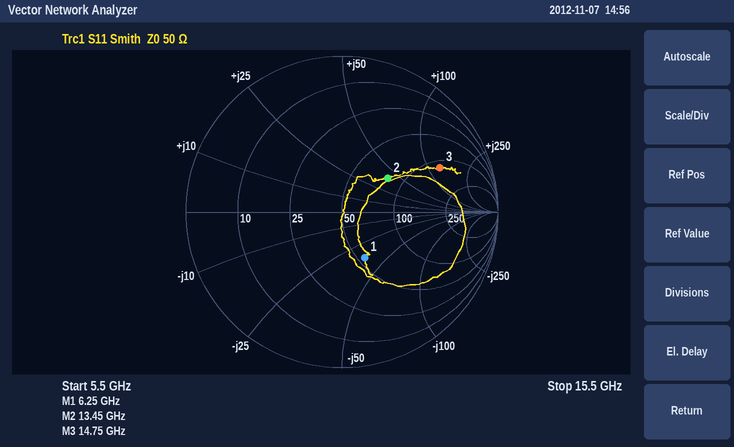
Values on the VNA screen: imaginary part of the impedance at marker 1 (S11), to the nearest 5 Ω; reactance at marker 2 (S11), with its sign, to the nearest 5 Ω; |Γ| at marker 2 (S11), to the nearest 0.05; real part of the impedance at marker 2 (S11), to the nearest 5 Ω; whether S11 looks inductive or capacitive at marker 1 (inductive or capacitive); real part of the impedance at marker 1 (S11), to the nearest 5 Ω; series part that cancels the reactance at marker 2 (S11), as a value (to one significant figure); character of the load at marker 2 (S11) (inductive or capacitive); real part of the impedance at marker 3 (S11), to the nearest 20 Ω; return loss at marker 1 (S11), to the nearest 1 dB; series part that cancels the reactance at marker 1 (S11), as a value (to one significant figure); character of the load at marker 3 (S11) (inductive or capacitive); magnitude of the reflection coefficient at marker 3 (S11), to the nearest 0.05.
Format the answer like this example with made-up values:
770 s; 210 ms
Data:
-35 Ω; +40 Ω; 0.35; 80 Ω; capacitive; 55 Ω; 300 fF; inductive; 120 Ω; 10 dB; 900 pH; inductive; 0.70
